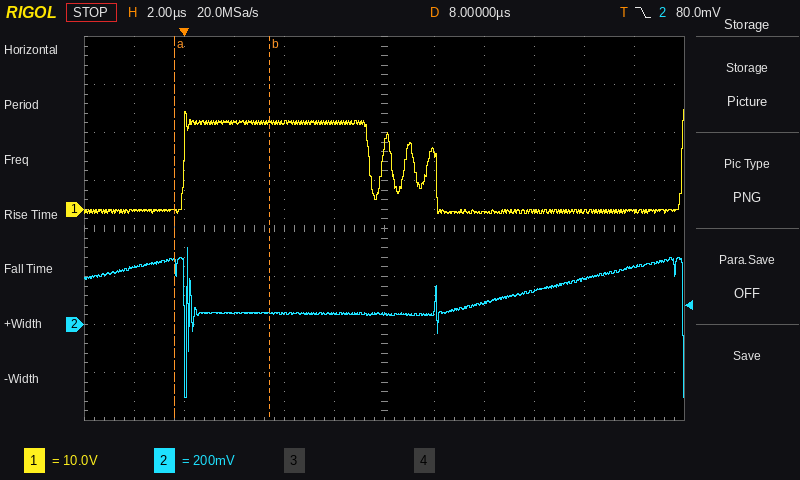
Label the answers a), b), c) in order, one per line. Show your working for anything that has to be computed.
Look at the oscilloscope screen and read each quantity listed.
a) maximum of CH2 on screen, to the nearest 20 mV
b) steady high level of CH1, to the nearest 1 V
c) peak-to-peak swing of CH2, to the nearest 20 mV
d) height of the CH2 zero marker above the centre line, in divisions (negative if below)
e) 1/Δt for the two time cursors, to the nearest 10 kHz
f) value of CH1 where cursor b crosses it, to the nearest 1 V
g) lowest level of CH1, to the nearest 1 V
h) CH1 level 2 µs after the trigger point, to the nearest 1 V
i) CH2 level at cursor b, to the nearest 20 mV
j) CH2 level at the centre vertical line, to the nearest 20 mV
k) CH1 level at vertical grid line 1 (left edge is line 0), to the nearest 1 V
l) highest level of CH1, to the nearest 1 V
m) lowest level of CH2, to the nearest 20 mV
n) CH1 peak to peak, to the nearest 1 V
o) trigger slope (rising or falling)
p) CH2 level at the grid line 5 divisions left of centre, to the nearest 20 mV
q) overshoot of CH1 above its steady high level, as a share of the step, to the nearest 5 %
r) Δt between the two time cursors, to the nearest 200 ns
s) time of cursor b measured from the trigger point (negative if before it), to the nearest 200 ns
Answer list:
a) 320 mV
b) 18 V
c) 320 mV − (-300 mV) = 620 mV
d) -2.0 div
e) 1 / 3.8 µs ≈ 260 kHz
f) 18 V
g) -1 V
h) 18 V
i) 40 mV
j) 40 mV
k) 0 V
l) 21 V
m) -300 mV
n) 21 V − (-1 V) = 22 V
o) falling
p) 240 mV
q) 15 %
r) 3.8 µs
s) +3.4 µs
